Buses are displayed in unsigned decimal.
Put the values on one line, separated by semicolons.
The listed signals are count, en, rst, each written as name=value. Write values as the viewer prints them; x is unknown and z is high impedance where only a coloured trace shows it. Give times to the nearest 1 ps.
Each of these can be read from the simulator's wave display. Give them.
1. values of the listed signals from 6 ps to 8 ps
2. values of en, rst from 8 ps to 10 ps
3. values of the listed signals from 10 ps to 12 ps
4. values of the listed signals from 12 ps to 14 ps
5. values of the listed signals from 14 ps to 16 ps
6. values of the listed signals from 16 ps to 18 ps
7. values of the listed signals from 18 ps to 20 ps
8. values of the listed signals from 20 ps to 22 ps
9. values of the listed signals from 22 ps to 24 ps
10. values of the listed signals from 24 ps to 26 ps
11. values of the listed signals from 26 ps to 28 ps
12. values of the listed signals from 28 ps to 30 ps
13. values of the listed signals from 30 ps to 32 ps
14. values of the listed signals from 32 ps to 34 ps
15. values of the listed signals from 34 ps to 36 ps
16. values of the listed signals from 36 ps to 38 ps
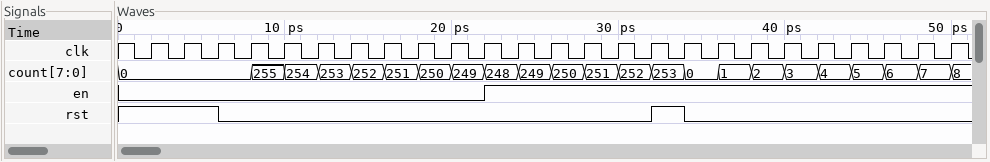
count=0, en=0, rst=0; en=0, rst=0; count=254, en=0, rst=0; count=253, en=0, rst=0; count=252, en=0, rst=0; count=251, en=0, rst=0; count=250, en=0, rst=0; count=249, en=0, rst=0; count=248, en=1, rst=0; count=249, en=1, rst=0; count=250, en=1, rst=0; count=251, en=1, rst=0; count=252, en=1, rst=0; count=253, en=1, rst=1; count=0, en=1, rst=0; count=1, en=1, rst=0
